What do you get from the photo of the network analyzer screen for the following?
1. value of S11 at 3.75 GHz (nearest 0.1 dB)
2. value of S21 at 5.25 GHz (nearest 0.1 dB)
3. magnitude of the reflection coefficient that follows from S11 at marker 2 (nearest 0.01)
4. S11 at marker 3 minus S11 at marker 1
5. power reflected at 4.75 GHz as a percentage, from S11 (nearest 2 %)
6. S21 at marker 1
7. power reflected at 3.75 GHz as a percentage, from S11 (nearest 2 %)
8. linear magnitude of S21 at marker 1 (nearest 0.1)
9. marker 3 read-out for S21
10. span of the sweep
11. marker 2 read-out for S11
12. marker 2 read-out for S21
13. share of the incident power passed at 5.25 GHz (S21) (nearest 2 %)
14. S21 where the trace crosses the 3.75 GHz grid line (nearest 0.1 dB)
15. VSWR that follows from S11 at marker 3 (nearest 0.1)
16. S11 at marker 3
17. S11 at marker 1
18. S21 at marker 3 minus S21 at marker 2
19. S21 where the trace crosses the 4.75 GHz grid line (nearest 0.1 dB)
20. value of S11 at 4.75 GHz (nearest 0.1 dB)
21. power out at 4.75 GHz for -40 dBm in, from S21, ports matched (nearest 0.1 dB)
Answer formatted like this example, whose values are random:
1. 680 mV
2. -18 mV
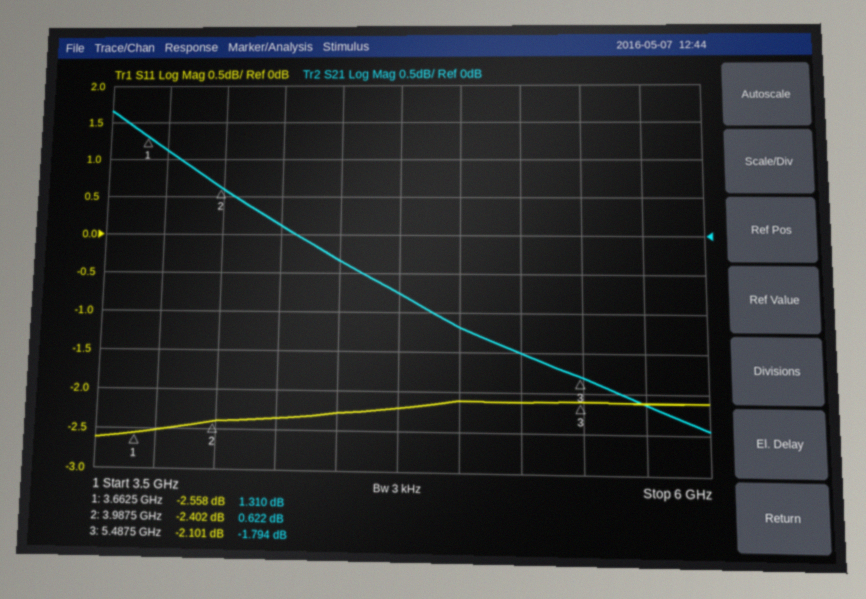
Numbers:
1. -2.5 dB
2. -1.5 dB
3. 0.76
4. 0.457 dB
5. 60 %
6. 1.310 dB
7. 56 %
8. 1.2
9. -1.794 dB
10. 2.5 GHz
11. -2.402 dB
12. 0.622 dB
13. 70 %
14. 1.1 dB
15. 8.3
16. -2.101 dB
17. -2.558 dB
18. -2.416 dB
19. -0.8 dB
20. -2.2 dB
21. -40.8 dBm
